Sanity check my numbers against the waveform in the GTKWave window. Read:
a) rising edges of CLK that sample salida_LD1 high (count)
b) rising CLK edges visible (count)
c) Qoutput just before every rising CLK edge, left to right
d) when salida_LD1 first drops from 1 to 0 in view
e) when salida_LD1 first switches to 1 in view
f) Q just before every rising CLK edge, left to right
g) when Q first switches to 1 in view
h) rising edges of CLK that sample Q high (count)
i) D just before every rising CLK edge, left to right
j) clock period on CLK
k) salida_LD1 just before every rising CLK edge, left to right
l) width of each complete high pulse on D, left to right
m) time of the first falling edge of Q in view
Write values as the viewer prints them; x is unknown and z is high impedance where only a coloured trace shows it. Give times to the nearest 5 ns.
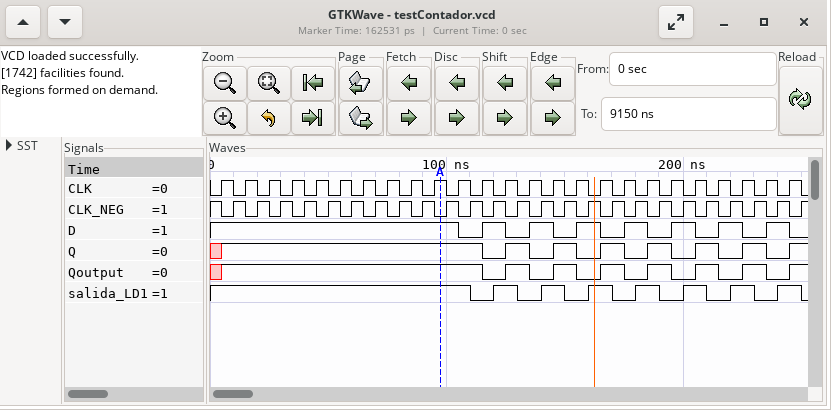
18
25
x 1 1 1 1 1 1 1 1 1 1 1 0 1 0 1 0 1 0 1 0 1 0 1 0
110 ns
120 ns
x 1 1 1 1 1 1 1 1 1 1 1 0 1 0 1 0 1 0 1 0 1 0 1 0
5 ns
17
1 1 1 1 1 1 1 1 1 1 1 0 1 0 1 0 1 0 1 0 1 0 1 0 1
10 ns
1 1 1 1 1 1 1 1 1 1 1 0 1 0 1 0 1 0 1 0 1 0 1 0 1
10 ns, 10 ns, 10 ns, 10 ns, 10 ns, 10 ns, 10 ns
115 ns
